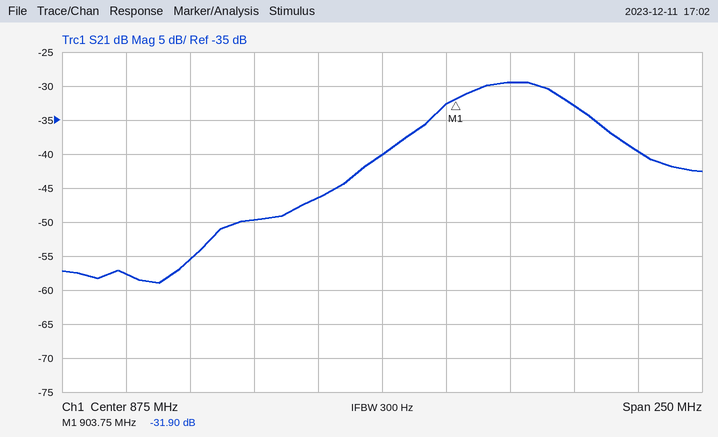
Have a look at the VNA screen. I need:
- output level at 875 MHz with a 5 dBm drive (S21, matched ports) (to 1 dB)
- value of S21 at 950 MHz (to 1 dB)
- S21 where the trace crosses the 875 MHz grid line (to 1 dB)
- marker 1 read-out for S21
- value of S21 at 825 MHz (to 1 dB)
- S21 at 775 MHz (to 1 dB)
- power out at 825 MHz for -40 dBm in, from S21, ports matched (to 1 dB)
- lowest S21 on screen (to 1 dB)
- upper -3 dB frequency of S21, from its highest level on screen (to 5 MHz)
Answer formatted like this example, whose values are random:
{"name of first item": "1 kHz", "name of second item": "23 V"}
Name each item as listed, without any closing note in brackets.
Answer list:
{"output level at 875 MHz with a 5 dBm drive (S21, matched ports)": "-35 dBm", "value of S21 at 950 MHz": "-33 dB", "S21 where the trace crosses the 875 MHz grid line": "-40 dB", "marker 1 read-out for S21": "-31.90 dB", "value of S21 at 825 MHz": "-50 dB", "S21 at 775 MHz": "-58 dB", "power out at 825 MHz for -40 dBm in, from S21, ports matched": "-90 dBm", "lowest S21 on screen": "-59 dB", "upper -3 dB frequency of S21, from its highest level on screen": "950 MHz"}
